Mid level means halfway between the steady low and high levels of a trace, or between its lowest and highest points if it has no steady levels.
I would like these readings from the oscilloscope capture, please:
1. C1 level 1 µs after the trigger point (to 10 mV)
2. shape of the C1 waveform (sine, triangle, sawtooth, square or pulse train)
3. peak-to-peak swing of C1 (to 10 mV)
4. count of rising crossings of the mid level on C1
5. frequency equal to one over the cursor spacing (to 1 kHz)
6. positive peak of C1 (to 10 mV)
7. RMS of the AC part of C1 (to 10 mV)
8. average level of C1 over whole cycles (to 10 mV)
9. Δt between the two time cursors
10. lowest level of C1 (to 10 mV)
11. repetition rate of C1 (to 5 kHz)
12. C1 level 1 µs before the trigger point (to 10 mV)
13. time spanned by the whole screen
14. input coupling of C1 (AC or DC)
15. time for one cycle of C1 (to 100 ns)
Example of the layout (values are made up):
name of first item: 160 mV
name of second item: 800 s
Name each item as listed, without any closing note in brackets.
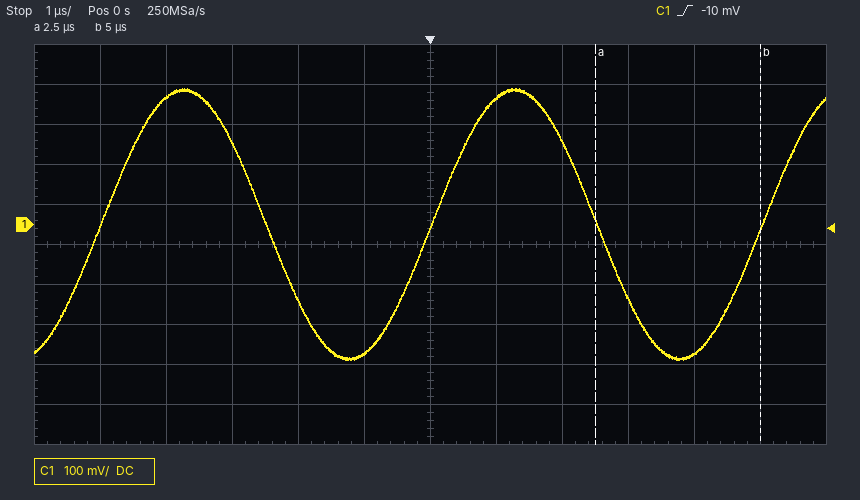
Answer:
C1 level 1 µs after the trigger point: 320 mV
shape of the C1 waveform: sine
peak-to-peak swing of C1: 680 mV
count of rising crossings of the mid level on C1: 3
frequency equal to one over the cursor spacing: 400 kHz
positive peak of C1: 340 mV
RMS of the AC part of C1: 240 mV
average level of C1 over whole cycles: 0 mV
Δt between the two time cursors: 2.5 µs
lowest level of C1: -340 mV
repetition rate of C1: 200 kHz
C1 level 1 µs before the trigger point: -320 mV
time spanned by the whole screen: 12 µs
input coupling of C1: DC
time for one cycle of C1: 5.0 µs
